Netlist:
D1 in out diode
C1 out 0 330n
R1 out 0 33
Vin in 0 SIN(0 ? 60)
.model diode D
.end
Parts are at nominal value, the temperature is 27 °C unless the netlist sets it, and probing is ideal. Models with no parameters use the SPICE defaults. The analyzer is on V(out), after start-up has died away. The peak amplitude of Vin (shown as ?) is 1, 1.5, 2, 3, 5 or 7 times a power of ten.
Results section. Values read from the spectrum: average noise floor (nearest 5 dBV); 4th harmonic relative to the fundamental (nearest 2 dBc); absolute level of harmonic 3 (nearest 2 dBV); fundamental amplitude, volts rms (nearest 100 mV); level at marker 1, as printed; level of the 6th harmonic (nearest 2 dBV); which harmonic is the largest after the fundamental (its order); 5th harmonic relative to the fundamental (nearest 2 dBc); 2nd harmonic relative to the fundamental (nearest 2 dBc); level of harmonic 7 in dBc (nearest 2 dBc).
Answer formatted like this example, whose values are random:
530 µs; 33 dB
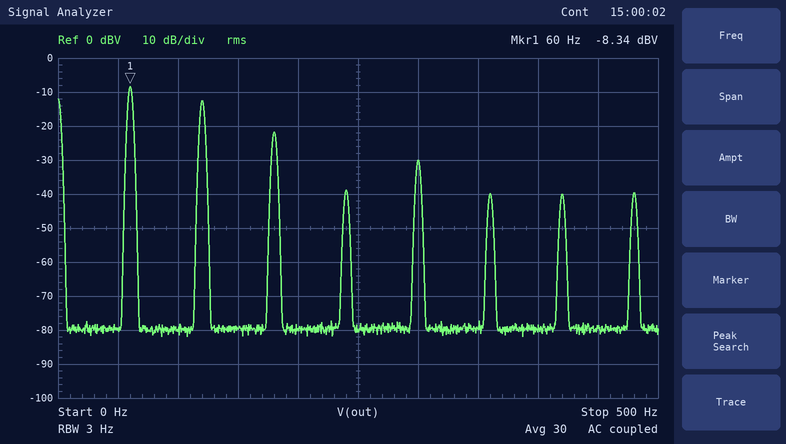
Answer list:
-80 dBV; -30 dBc; -22 dBV; 400 mV; -8.34 dBV; -40 dBV; 2; -22 dBc; -4 dBc; -32 dBc
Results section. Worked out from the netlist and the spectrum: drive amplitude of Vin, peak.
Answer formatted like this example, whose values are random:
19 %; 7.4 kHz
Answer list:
2 V
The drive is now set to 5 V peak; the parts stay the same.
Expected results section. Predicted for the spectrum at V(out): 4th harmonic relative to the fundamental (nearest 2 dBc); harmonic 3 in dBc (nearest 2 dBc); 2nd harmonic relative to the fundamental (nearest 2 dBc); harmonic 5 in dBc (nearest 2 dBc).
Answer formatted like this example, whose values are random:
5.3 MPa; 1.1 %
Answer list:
-22 dBc; -22 dBc; -6 dBc; -28 dBc
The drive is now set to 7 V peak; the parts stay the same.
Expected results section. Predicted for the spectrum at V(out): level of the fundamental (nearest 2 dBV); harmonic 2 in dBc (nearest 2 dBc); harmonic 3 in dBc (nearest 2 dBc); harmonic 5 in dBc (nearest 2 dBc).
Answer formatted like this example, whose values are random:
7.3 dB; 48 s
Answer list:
6 dBV; -6 dBc; -26 dBc; -30 dBc
